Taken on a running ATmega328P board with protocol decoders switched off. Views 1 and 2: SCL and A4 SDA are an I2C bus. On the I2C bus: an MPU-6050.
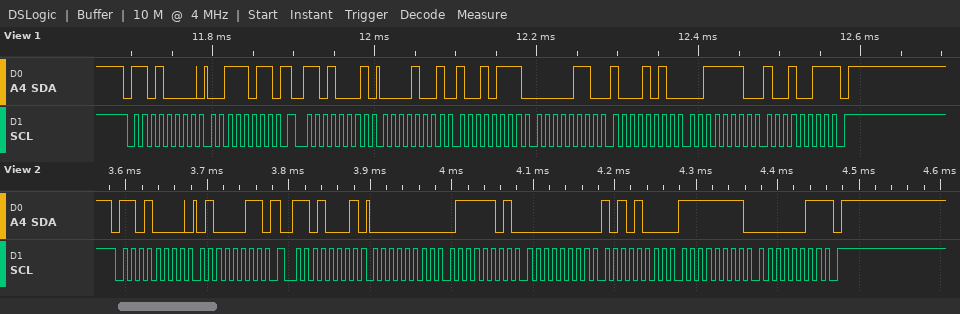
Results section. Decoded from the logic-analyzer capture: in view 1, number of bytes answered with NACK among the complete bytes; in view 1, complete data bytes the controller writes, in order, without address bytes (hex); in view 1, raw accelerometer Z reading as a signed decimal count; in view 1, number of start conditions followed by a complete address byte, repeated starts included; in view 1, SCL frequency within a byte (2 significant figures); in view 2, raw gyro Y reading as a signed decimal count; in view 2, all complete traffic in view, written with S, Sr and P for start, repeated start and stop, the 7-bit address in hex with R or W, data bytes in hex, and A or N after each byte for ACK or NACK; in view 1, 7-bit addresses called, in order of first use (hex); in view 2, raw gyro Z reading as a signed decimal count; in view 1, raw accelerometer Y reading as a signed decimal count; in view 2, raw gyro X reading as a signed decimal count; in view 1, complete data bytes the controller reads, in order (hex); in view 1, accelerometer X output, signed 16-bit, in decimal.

1
3B
16019
2
100 kHz
168
S 68W A 43 A Sr 68R A 00 A 7D A 00 A A8 A FF A 03 N P
0x68
-253
1674
125
09 97 06 8A 3E 93
2455
